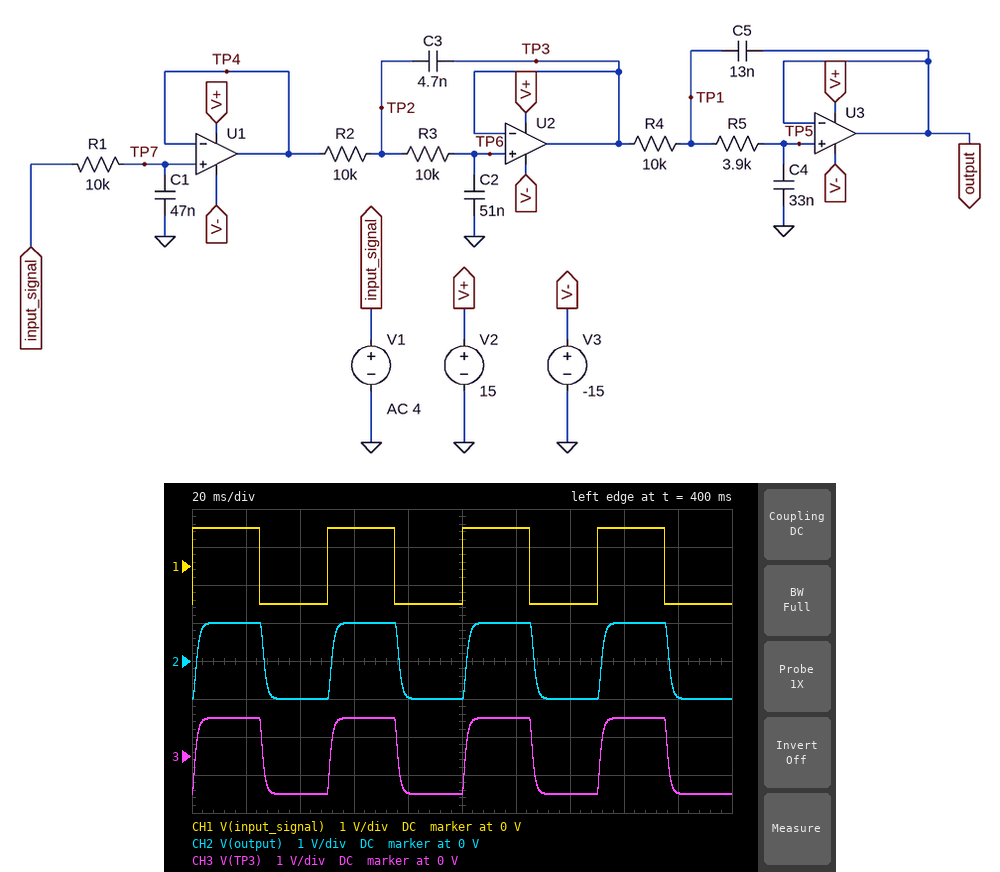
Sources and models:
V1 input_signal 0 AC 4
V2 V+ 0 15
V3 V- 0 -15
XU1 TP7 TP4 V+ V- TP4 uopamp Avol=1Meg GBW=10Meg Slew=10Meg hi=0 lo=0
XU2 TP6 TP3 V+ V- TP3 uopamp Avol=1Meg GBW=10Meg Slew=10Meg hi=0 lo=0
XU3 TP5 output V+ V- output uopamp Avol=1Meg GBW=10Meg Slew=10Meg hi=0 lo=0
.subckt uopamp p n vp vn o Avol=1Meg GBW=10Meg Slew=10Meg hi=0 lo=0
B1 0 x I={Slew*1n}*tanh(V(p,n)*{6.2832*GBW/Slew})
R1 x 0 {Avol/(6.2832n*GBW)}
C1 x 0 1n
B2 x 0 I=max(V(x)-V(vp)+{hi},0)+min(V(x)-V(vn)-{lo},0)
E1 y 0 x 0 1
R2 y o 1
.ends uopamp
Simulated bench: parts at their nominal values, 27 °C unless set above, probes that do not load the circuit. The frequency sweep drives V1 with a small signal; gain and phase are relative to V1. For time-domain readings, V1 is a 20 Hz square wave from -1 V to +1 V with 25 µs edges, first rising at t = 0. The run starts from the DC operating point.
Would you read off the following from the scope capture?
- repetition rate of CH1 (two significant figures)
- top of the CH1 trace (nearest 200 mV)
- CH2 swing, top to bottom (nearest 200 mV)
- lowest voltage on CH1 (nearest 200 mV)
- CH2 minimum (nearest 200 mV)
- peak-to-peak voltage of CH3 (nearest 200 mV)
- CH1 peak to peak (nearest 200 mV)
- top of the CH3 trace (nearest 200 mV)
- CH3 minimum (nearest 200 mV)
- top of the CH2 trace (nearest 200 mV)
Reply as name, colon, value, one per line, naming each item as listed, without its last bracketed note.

repetition rate of CH1: 20 Hz
top of the CH1 trace: 1.0 V
CH2 swing, top to bottom: 2.0 V
lowest voltage on CH1: -1.0 V
CH2 minimum: -1.0 V
peak-to-peak voltage of CH3: 2.0 V
CH1 peak to peak: 2.0 V
top of the CH3 trace: 1.0 V
CH3 minimum: -1.0 V
top of the CH2 trace: 1.0 V
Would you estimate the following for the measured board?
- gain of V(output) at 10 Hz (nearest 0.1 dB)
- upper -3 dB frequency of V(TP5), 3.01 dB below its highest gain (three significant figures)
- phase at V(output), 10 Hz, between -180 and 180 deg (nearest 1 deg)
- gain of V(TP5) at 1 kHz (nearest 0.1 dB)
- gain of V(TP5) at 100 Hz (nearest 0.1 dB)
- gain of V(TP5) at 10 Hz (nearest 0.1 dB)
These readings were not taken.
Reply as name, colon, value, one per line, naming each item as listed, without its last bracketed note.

gain of V(output) at 10 Hz: 0 dB
upper -3 dB frequency of V(TP5), 3.01 dB below its highest gain: 123 Hz
phase at V(output), 10 Hz, between -180 and 180 deg: -7 deg
gain of V(TP5) at 1 kHz: -35.3 dB
gain of V(TP5) at 100 Hz: -2.1 dB
gain of V(TP5) at 10 Hz: 0 dB
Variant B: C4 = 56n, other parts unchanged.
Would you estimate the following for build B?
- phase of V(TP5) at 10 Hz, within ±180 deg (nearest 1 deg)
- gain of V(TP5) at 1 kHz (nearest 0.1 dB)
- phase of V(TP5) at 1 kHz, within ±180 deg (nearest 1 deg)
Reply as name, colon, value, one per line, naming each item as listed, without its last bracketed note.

phase of V(TP5) at 10 Hz, within ±180 deg: -8 deg
gain of V(TP5) at 1 kHz: -39.8 dB
phase of V(TP5) at 1 kHz, within ±180 deg: 108 deg
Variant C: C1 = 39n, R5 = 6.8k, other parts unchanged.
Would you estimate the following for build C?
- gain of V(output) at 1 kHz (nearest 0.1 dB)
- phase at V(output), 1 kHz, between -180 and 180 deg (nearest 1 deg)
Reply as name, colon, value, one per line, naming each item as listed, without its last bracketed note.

gain of V(output) at 1 kHz: -35.4 dB
phase at V(output), 1 kHz, between -180 and 180 deg: 110 deg
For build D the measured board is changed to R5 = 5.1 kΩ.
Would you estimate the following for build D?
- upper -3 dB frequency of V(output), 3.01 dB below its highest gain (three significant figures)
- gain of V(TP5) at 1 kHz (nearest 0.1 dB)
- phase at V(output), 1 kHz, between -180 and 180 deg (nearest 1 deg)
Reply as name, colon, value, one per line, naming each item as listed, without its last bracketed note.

upper -3 dB frequency of V(output), 3.01 dB below its highest gain: 122 Hz
gain of V(TP5) at 1 kHz: -35.9 dB
phase at V(output), 1 kHz, between -180 and 180 deg: 112 deg
